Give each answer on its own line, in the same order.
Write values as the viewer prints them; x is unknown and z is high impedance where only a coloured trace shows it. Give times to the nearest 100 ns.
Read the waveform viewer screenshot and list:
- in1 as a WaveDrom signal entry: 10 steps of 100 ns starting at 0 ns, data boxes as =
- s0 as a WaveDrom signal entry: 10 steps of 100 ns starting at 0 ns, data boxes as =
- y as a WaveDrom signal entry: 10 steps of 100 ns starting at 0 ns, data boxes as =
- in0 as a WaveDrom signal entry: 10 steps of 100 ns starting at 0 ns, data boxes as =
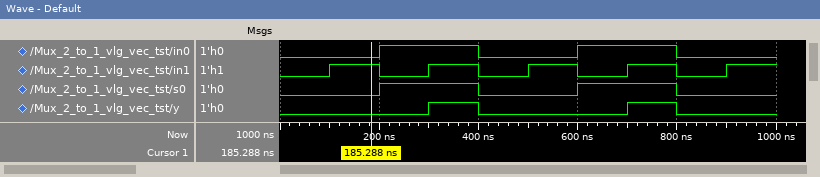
{name: 'in1', wave: '0101010101'}
{name: 's0', wave: '0.1.0.1.0.'}
{name: 'y', wave: '0..10..10.'}
{name: 'in0', wave: '0.1.0.1.0.'}
